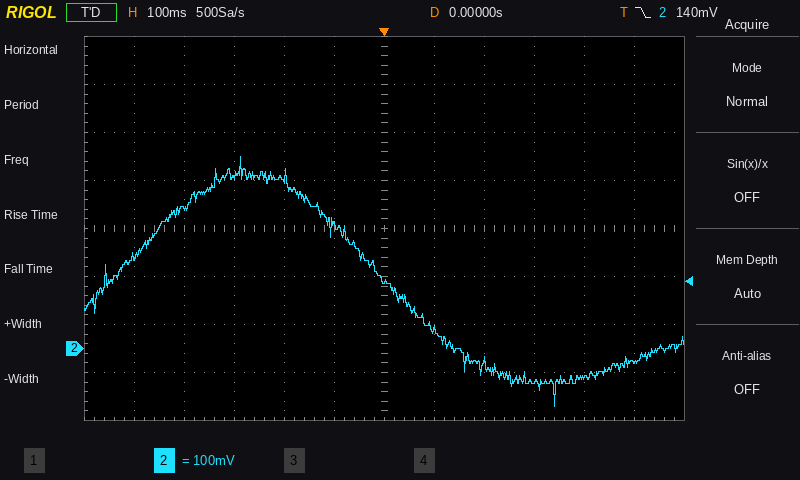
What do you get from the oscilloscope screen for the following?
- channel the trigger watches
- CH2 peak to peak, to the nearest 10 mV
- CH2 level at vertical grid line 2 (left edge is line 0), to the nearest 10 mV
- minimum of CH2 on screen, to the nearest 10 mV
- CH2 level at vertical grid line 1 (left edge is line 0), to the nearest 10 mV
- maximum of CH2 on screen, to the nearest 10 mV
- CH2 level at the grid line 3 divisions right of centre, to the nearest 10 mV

CH2
520 mV
290 mV
-120 mV
190 mV
400 mV
-70 mV
